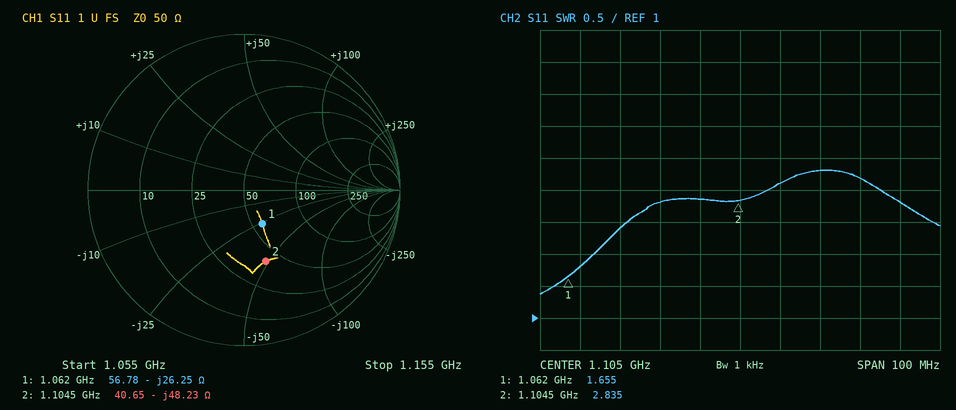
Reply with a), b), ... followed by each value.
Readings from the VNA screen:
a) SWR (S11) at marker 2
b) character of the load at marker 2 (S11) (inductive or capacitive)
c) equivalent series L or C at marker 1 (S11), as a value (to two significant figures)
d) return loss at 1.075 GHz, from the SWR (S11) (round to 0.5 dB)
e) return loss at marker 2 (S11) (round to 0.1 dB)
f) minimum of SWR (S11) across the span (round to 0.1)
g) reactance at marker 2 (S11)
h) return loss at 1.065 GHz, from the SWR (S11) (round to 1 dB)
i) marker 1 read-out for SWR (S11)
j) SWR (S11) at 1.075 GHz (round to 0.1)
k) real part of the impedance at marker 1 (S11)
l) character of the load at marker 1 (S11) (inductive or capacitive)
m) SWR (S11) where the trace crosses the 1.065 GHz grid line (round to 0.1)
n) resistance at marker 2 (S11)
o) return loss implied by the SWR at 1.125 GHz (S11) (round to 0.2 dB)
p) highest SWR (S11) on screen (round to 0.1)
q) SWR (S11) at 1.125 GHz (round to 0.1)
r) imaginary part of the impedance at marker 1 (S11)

a) 2.835
b) capacitive
c) 5.7 pF
d) 7.5 dB
e) 6.4 dB
f) 1.4
g) -48.23 Ω
h) 11 dB
i) 1.655
j) 2.4
k) 56.78 Ω
l) capacitive
m) 1.8
n) 40.65 Ω
o) 5.4 dB
p) 3.3
q) 3.3
r) -26.25 Ω
